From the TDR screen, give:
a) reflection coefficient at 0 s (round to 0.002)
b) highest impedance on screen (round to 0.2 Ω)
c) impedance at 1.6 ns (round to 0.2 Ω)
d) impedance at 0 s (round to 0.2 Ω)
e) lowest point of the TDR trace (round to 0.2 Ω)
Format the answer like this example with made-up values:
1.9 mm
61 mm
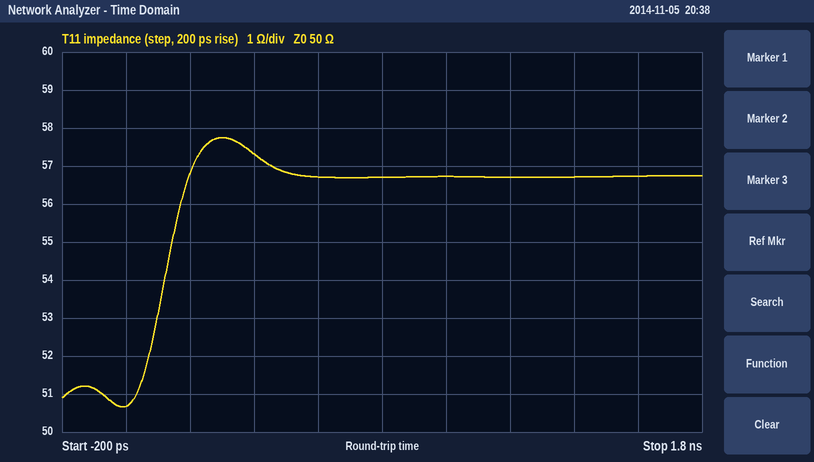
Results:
+0.006
57.8 Ω
56.8 Ω
50.6 Ω
50.6 Ω
